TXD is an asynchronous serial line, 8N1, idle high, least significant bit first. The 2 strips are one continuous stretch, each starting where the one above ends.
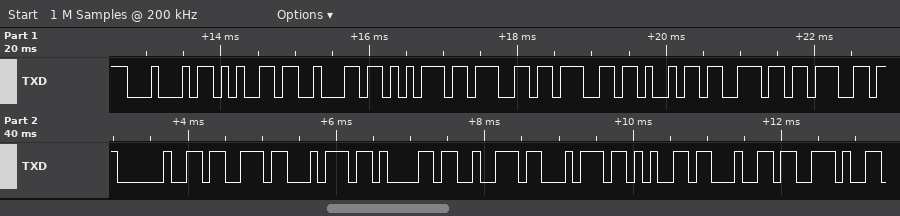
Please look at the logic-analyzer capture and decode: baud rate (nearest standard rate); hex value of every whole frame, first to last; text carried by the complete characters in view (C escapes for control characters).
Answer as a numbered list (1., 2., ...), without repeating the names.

1. 9600 baud
2. 44 65 62 75 67 67 69 6E 67 20 73 74 61 72 74 65 64 2E
3. "Debugging started."
